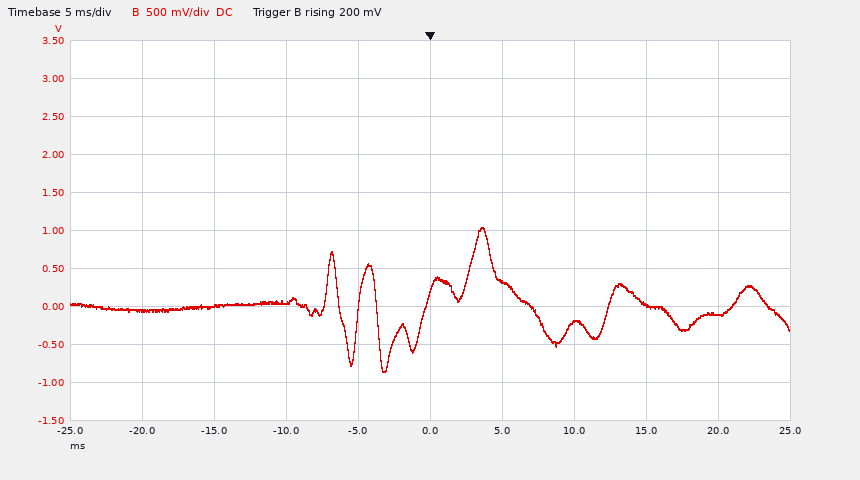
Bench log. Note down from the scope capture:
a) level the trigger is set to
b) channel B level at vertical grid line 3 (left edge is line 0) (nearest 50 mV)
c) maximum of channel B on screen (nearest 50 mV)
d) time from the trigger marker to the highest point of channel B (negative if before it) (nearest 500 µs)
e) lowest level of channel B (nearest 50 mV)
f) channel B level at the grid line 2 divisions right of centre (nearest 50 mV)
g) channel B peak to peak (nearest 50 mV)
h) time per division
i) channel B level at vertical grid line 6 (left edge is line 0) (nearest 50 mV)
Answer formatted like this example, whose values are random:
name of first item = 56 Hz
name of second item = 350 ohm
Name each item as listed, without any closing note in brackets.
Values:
level the trigger is set to = 200 mV
channel B level at vertical grid line 3 (left edge is line 0) = 50 mV
maximum of channel B on screen = 1.05 V
time from the trigger marker to the highest point of channel B (negative if before it) = +3.5 ms
lowest level of channel B = -850 mV
channel B level at the grid line 2 divisions right of centre = -200 mV
channel B peak to peak = 1.90 V
time per division = 5 ms
channel B level at vertical grid line 6 (left edge is line 0) = 350 mV
